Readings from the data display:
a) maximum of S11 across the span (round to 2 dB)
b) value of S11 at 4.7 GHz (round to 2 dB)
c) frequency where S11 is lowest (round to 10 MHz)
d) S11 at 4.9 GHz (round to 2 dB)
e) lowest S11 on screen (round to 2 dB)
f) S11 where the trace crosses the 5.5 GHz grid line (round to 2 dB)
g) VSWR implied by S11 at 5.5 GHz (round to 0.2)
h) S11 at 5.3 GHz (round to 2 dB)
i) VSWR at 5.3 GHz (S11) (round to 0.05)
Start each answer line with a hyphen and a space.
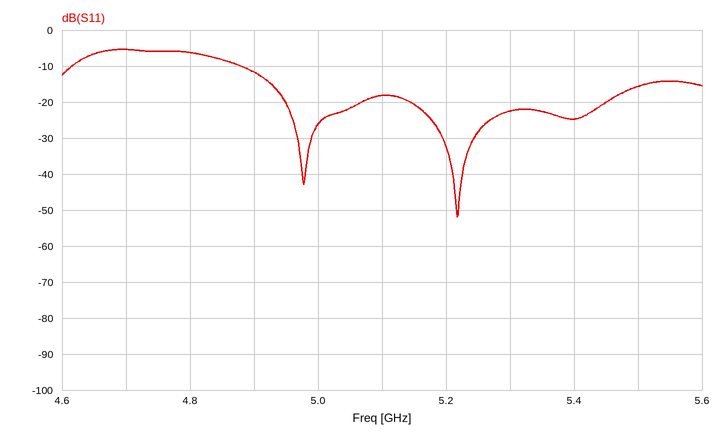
- -6 dB
- -6 dB
- 5.22 GHz
- -12 dB
- -52 dB
- -16 dB
- 1.4
- -22 dB
- 1.15
